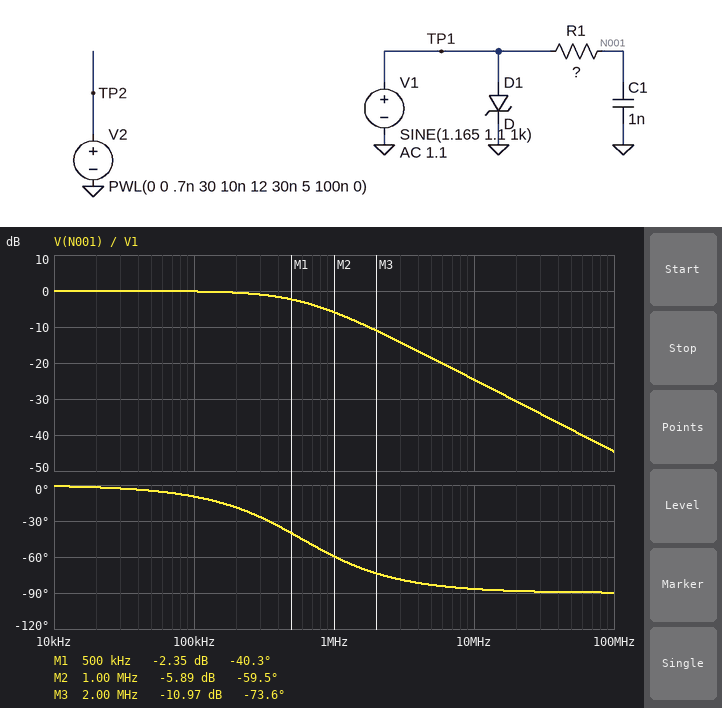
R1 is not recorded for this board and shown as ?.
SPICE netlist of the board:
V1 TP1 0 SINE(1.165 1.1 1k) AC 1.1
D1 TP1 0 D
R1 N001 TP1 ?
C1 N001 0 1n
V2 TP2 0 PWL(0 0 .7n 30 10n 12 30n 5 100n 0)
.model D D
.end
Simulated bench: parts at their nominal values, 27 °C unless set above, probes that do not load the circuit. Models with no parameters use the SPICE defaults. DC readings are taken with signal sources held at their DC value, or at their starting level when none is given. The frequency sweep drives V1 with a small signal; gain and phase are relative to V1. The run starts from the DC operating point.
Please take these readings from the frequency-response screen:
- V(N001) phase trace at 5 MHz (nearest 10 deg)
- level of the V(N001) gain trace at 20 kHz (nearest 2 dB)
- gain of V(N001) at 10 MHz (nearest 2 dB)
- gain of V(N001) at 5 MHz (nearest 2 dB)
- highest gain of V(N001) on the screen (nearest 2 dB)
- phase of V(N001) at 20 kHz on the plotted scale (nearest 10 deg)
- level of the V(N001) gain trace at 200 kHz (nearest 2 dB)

-80 deg
0 dB
-24 dB
-18 dB
0 dB
0 deg
0 dB
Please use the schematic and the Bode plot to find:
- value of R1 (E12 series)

270 Ω
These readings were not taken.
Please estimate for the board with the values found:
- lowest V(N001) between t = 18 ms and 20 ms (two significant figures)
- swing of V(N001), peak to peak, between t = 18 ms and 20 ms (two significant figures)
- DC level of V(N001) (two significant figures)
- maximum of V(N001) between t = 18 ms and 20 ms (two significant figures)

65 mV
2.2 V
1.2 V
2.3 V
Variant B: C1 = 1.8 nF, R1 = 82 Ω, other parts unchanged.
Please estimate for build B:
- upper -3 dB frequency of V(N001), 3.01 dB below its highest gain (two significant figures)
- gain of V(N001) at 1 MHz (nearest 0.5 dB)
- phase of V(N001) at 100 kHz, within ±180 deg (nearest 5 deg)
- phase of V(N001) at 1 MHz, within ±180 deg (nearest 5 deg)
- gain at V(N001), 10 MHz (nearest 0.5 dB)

1.1 MHz
-2.5 dB
-5 deg
-45 deg
-19.5 dB
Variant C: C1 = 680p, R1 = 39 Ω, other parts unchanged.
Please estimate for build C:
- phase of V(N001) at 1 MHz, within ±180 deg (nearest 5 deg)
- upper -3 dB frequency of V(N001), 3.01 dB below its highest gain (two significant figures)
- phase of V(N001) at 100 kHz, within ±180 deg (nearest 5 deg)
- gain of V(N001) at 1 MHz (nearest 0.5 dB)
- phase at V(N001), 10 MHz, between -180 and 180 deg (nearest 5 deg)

-10 deg
6.0 MHz
0 deg
0 dB
-60 deg
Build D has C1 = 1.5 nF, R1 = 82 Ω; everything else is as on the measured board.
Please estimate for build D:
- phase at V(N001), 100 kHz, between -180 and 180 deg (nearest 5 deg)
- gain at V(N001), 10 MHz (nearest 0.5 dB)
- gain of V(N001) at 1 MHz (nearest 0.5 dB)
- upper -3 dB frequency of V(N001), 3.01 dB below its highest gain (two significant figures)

-5 deg
-18.0 dB
-2.0 dB
1.3 MHz
